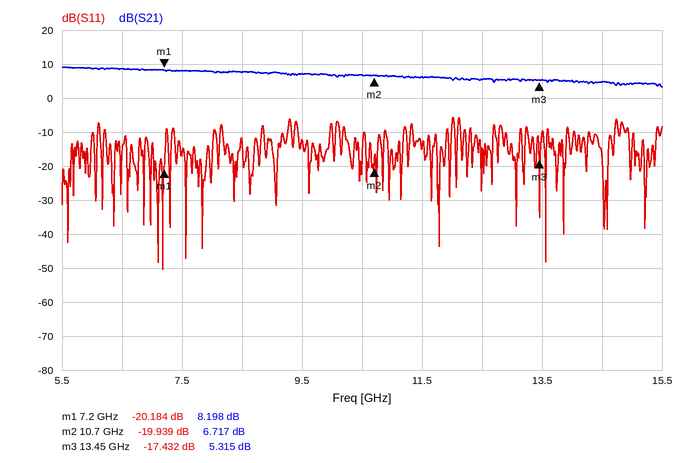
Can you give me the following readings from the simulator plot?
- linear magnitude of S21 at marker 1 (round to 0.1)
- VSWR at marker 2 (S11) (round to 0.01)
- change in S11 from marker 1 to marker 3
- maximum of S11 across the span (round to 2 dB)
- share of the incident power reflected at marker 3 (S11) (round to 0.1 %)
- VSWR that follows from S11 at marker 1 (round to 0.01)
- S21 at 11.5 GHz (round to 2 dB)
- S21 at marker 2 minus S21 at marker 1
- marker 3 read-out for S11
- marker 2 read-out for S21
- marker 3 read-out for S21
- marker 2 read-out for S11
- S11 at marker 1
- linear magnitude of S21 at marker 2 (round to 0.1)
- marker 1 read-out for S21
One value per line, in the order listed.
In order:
2.6
1.22
2.752 dB
-6 dB
1.8 %
1.22
6 dB
-1.481 dB
-17.432 dB
6.717 dB
5.315 dB
-19.939 dB
-20.184 dB
2.2
8.198 dB
